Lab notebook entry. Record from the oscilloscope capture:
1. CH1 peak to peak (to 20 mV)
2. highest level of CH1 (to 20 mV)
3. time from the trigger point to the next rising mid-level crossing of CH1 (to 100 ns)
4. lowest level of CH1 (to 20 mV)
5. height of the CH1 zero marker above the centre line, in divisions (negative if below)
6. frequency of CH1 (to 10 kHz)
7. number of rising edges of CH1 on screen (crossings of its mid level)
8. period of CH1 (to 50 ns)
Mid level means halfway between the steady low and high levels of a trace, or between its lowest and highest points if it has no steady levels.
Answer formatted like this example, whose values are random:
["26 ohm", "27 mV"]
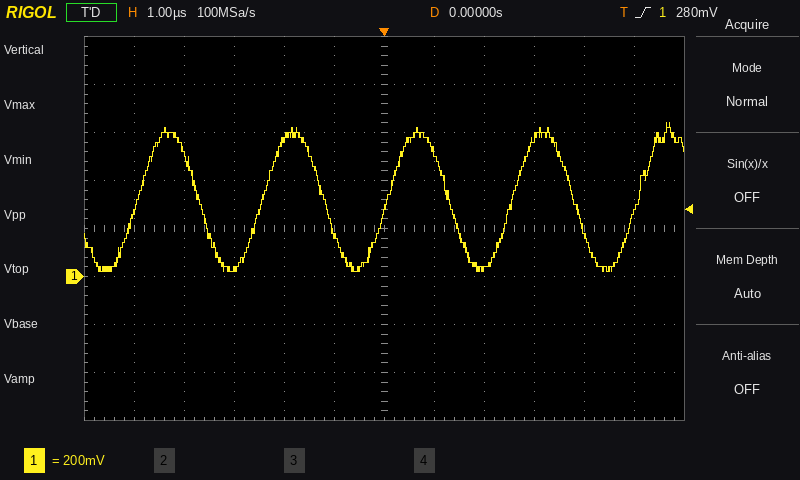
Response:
["620 mV", "640 mV", "100 ns", "20 mV", "-1.0 div", "400 kHz", "5", "2.50 µs"]
